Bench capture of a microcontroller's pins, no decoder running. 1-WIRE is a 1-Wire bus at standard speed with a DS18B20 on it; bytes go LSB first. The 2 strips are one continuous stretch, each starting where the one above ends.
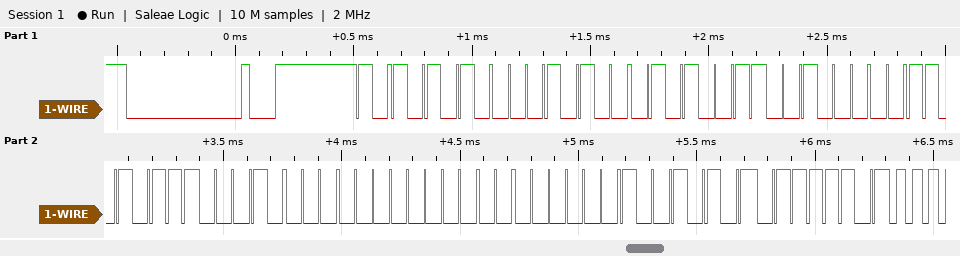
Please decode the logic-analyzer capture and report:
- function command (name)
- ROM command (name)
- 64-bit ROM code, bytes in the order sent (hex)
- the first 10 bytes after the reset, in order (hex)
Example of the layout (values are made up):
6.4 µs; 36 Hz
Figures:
Read Scratchpad; Match ROM; 28 CA 04 EB 08 00 00 A9; 55 28 CA 04 EB 08 00 00 A9 BE
